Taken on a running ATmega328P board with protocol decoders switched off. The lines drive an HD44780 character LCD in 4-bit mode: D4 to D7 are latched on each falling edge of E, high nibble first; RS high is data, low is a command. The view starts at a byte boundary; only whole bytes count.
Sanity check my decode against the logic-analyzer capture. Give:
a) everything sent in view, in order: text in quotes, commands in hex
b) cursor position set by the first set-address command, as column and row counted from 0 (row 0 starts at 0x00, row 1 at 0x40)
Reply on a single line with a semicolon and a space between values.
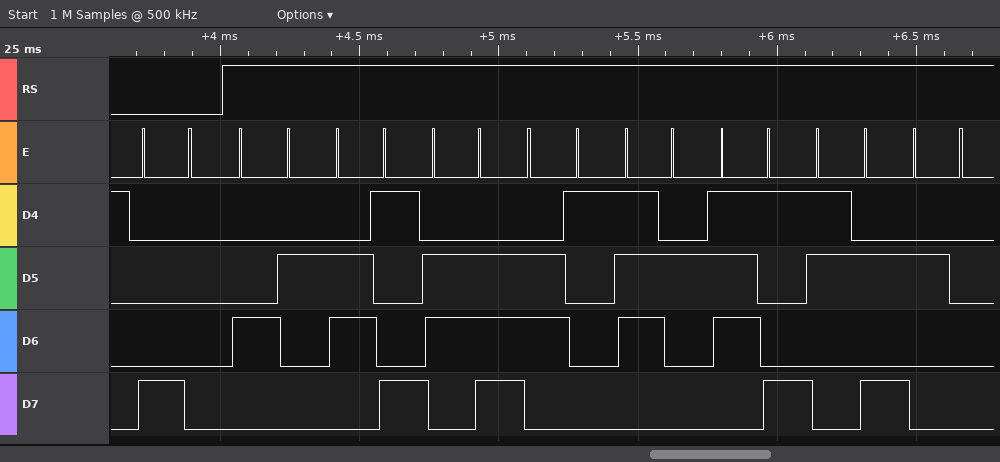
0x80 "Binary: "; column 0, row 0
